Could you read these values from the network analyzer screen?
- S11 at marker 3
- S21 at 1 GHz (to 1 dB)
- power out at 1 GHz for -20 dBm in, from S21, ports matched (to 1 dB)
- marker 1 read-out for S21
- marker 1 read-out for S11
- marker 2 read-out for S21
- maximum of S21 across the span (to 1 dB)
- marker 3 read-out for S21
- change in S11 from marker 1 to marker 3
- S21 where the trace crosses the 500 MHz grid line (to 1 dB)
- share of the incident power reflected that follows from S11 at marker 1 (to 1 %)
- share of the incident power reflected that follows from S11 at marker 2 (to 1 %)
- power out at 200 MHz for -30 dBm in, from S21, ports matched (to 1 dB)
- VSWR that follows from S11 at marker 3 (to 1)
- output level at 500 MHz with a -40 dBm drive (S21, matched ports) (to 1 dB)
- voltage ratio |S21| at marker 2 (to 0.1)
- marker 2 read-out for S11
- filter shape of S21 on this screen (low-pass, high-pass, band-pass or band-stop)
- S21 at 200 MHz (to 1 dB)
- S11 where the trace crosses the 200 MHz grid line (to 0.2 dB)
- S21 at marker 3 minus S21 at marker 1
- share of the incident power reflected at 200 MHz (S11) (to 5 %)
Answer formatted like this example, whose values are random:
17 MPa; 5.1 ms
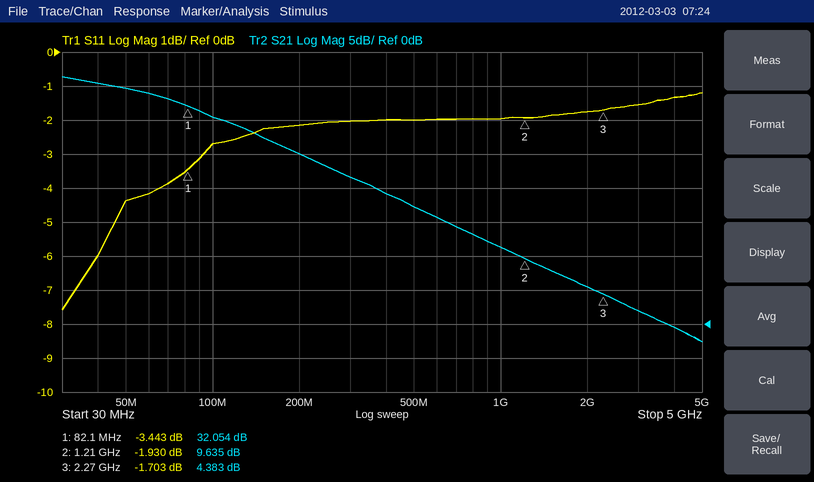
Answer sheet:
-1.703 dB; 11 dB; -9 dBm; 32.054 dB; -3.443 dB; 9.635 dB; 36 dB; 4.383 dB; 1.740 dB; 17 dB; 45 %; 64 %; -5 dBm; 10; -23 dBm; 3.0; -1.930 dB; low-pass; 25 dB; -2.2 dB; -27.671 dB; 60 %
